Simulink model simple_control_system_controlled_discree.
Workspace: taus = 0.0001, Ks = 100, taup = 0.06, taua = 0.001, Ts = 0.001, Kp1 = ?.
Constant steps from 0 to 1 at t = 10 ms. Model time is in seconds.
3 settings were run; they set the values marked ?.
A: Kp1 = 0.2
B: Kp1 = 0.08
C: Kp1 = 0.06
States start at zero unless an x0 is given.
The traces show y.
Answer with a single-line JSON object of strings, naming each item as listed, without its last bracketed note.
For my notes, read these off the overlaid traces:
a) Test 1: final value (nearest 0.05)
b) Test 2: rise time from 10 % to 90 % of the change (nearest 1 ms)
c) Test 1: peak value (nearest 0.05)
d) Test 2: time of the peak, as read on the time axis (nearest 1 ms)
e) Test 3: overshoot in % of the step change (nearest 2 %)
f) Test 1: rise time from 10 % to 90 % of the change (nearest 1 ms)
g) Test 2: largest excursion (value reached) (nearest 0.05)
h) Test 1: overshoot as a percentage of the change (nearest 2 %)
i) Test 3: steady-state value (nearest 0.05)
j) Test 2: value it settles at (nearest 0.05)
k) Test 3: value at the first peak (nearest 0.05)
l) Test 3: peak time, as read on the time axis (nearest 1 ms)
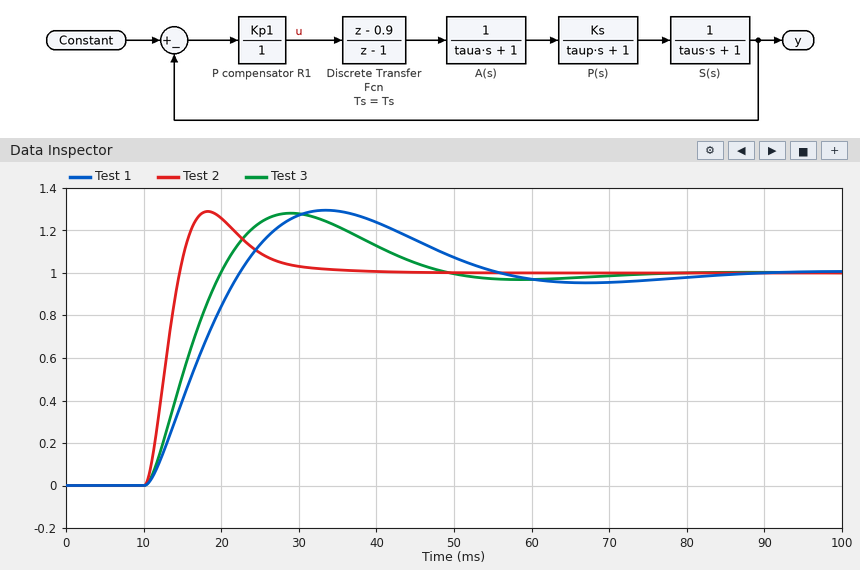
{"Test 1: final value": "1.00", "Test 2: rise time from 10 % to 90 % of the change": "3 ms", "Test 1: peak value": "1.30", "Test 2: time of the peak, as read on the time axis": "18 ms", "Test 3: overshoot in % of the step change": "28 %", "Test 1: rise time from 10 % to 90 % of the change": "9 ms", "Test 2: largest excursion (value reached)": "1.30", "Test 1: overshoot as a percentage of the change": "30 %", "Test 3: steady-state value": "1.00", "Test 2: value it settles at": "1.00", "Test 3: value at the first peak": "1.30", "Test 3: peak time, as read on the time axis": "29 ms"}
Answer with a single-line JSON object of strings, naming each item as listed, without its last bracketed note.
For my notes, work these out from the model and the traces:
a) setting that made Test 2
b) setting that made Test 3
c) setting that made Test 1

{"setting that made Test 2": "A", "setting that made Test 3": "B", "setting that made Test 1": "C"}
